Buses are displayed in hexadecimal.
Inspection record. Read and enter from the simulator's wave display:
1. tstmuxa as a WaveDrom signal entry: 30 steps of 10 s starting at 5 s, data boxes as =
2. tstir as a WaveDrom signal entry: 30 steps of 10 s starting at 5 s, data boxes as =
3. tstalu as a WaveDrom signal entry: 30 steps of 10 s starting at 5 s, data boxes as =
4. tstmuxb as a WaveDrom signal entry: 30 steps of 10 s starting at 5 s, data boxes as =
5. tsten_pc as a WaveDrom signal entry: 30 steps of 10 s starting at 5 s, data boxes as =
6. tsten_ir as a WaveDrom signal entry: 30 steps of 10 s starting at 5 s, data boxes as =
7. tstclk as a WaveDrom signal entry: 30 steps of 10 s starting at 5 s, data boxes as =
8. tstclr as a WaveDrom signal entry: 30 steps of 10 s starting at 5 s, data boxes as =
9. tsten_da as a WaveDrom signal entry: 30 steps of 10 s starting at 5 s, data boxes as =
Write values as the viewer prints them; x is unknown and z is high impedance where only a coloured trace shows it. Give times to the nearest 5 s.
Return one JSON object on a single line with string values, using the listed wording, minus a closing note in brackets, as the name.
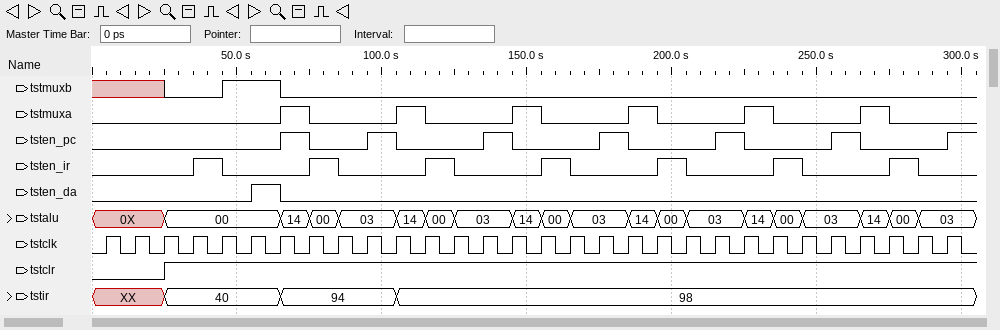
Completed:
{"tstmuxa as a WaveDrom signal entry: 30 steps of 10 s starting at 5 s, data boxes as =": "{name: 'tstmuxa', wave: '0.....10..10..10..10..10..10..'}", "tstir as a WaveDrom signal entry: 30 steps of 10 s starting at 5 s, data boxes as =": "{name: 'tstir', wave: 'x.=...=...=...................', data: '40 94 98'}", "tstalu as a WaveDrom signal entry: 30 steps of 10 s starting at 5 s, data boxes as =": "{name: 'tstalu', wave: '=.=...===.===.===.===.===.===.', data: '0X 00 14 00 03 14 00 03 14 00 03 14 00 03 14 00 03 14 00 03'}", "tstmuxb as a WaveDrom signal entry: 30 steps of 10 s starting at 5 s, data boxes as =": "{name: 'tstmuxb', wave: 'x.0.1.0.......................'}", "tsten_pc as a WaveDrom signal entry: 30 steps of 10 s starting at 5 s, data boxes as =": "{name: 'tsten_pc', wave: '0.....10.10..10..10..10..10..1'}", "tsten_ir as a WaveDrom signal entry: 30 steps of 10 s starting at 5 s, data boxes as =": "{name: 'tsten_ir', wave: '0..10..10..10..10..10..10..10.'}", "tstclk as a WaveDrom signal entry: 30 steps of 10 s starting at 5 s, data boxes as =": "{name: 'tstclk', wave: 'p.............................'}", "tstclr as a WaveDrom signal entry: 30 steps of 10 s starting at 5 s, data boxes as =": "{name: 'tstclr', wave: '0.1...........................'}", "tsten_da as a WaveDrom signal entry: 30 steps of 10 s starting at 5 s, data boxes as =": "{name: 'tsten_da', wave: '0....10.......................'}"}
